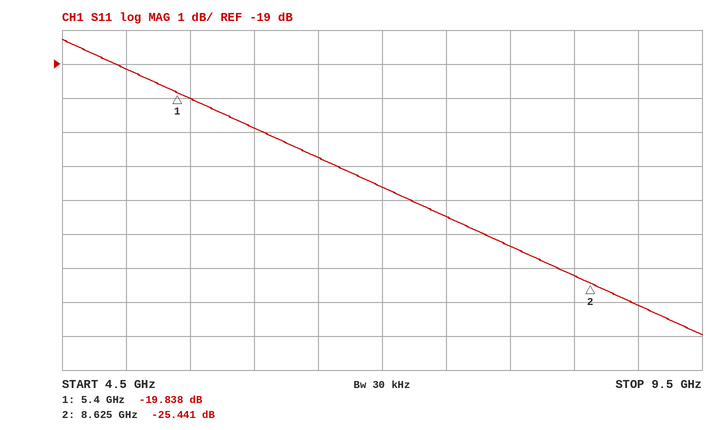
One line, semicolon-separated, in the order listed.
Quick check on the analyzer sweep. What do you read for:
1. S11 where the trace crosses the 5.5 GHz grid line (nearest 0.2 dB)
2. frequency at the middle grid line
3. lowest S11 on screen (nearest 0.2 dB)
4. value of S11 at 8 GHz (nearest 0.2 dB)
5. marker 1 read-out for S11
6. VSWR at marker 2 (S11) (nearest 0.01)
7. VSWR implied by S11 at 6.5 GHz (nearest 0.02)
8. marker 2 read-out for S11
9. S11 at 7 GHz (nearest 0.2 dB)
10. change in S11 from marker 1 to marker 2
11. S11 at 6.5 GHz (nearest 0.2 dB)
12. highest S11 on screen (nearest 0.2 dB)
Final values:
-20.0 dB; 7 GHz; -27.0 dB; -24.4 dB; -19.838 dB; 1.11; 1.18; -25.441 dB; -22.6 dB; -5.603 dB; -21.8 dB; -18.2 dB
